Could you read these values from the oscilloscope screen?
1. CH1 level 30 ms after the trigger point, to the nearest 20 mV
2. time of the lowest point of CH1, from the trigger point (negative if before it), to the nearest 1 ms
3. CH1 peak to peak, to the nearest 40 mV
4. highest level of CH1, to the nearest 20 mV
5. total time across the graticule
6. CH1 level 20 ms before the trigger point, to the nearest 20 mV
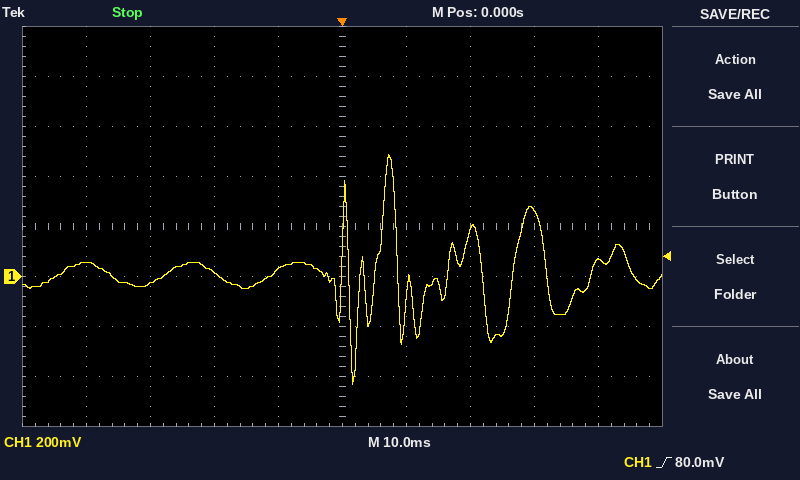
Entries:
260 mV
+2 ms
920 mV
480 mV
100 ms
20 mV
